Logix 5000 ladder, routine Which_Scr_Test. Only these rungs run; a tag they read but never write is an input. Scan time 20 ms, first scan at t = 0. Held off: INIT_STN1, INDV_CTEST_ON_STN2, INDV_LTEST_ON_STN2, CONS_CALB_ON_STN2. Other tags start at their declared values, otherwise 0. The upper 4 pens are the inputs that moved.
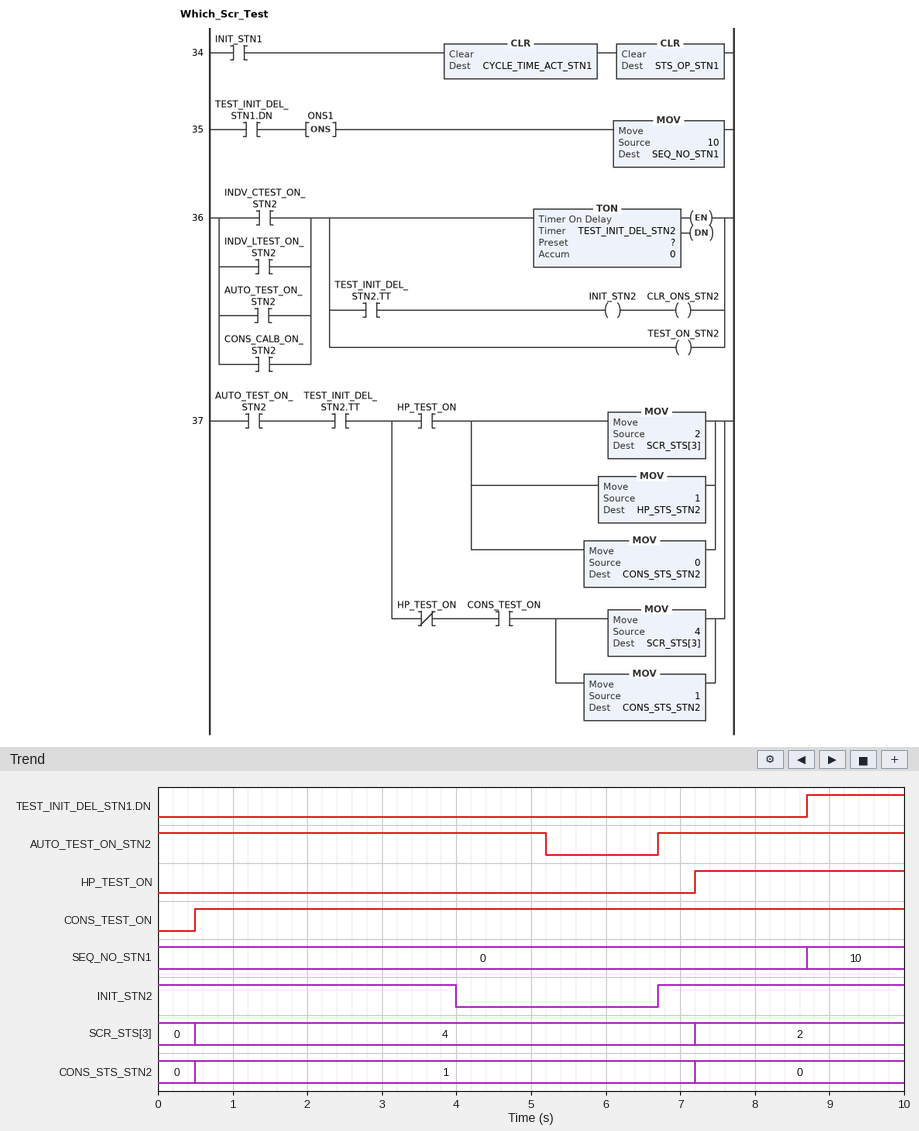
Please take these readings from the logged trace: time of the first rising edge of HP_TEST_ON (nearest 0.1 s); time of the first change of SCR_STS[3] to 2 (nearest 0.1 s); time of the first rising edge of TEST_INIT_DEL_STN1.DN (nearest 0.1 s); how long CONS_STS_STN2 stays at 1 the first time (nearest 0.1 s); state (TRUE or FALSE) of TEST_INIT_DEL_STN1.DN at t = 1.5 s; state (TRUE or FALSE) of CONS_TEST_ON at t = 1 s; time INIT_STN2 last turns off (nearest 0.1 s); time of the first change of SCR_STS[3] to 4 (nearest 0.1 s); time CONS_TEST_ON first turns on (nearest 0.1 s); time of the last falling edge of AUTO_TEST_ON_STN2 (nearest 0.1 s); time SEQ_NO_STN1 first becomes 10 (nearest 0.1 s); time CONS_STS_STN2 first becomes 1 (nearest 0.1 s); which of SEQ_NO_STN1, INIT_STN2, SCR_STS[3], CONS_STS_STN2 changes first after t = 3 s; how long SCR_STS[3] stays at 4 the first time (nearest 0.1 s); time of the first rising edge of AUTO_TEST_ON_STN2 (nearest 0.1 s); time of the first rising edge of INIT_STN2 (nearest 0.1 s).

7.2 s
7.2 s
8.7 s
6.7 s
FALSE
TRUE
4.0 s
0.5 s
0.5 s
5.2 s
8.7 s
0.5 s
INIT_STN2
6.7 s
6.7 s
6.7 s
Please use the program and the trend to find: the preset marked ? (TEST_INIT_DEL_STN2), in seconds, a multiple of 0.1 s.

4.0 s
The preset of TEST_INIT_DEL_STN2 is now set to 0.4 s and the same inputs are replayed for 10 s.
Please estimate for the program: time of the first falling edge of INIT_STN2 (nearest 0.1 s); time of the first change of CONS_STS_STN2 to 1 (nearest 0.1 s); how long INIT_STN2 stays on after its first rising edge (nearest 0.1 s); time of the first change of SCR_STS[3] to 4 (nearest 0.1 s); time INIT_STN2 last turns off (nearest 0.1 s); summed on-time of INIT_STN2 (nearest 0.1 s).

0.4 s
6.7 s
0.4 s
6.7 s
7.1 s
0.8 s
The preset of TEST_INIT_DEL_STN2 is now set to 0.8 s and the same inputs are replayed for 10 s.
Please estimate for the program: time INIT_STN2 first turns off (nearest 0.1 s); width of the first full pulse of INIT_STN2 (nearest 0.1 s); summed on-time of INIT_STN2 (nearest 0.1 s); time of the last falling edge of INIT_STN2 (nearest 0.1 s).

0.8 s
0.8 s
1.6 s
7.5 s
